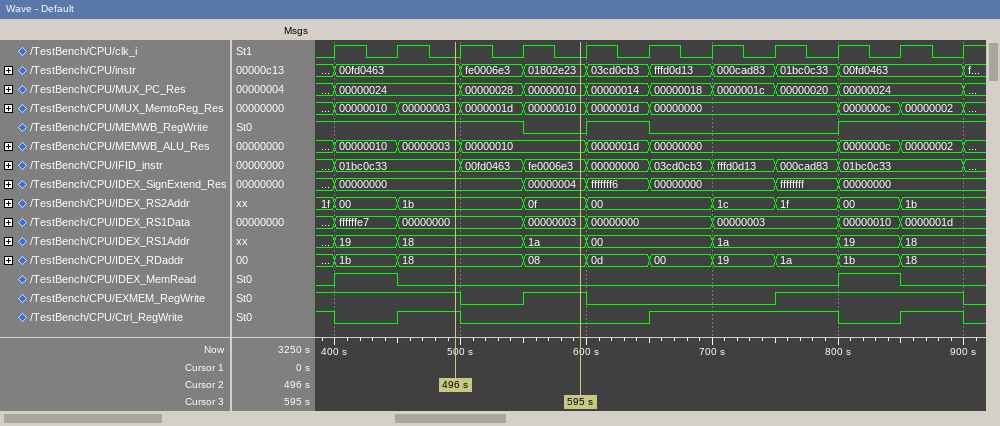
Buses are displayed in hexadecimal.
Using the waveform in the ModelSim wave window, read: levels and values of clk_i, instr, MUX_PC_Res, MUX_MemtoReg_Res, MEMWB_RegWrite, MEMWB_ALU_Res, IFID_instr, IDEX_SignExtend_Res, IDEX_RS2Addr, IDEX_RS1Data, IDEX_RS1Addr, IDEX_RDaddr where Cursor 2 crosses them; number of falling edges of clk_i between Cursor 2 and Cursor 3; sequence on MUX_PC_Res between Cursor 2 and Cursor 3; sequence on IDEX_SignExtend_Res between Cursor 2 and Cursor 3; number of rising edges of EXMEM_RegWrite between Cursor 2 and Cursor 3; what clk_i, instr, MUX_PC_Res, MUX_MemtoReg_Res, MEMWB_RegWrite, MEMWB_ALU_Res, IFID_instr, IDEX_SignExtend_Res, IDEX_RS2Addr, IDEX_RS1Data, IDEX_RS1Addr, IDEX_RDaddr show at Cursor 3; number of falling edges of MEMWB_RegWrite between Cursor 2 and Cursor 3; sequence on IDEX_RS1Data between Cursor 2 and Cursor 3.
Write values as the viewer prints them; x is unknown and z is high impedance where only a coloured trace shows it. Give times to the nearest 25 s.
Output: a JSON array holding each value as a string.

["clk_i=0, instr=00fd0463, MUX_PC_Res=00000024, MUX_MemtoReg_Res=00000003, MEMWB_RegWrite=1, MEMWB_ALU_Res=00000003, IFID_instr=01bc0c33, IDEX_SignExtend_Res=00000000, IDEX_RS2Addr=1b, IDEX_RS1Data=00000000, IDEX_RS1Addr=18, IDEX_RDaddr=18", "2", "00000024, 00000028, 00000010", "00000000, 00000004", "1", "clk_i=0, instr=01802e23, MUX_PC_Res=00000010, MUX_MemtoReg_Res=00000010, MEMWB_RegWrite=0, MEMWB_ALU_Res=00000010, IFID_instr=fe0006e3, IDEX_SignExtend_Res=00000004, IDEX_RS2Addr=0f, IDEX_RS1Data=00000003, IDEX_RS1Addr=1a, IDEX_RDaddr=08", "1", "00000000, 00000003"]
